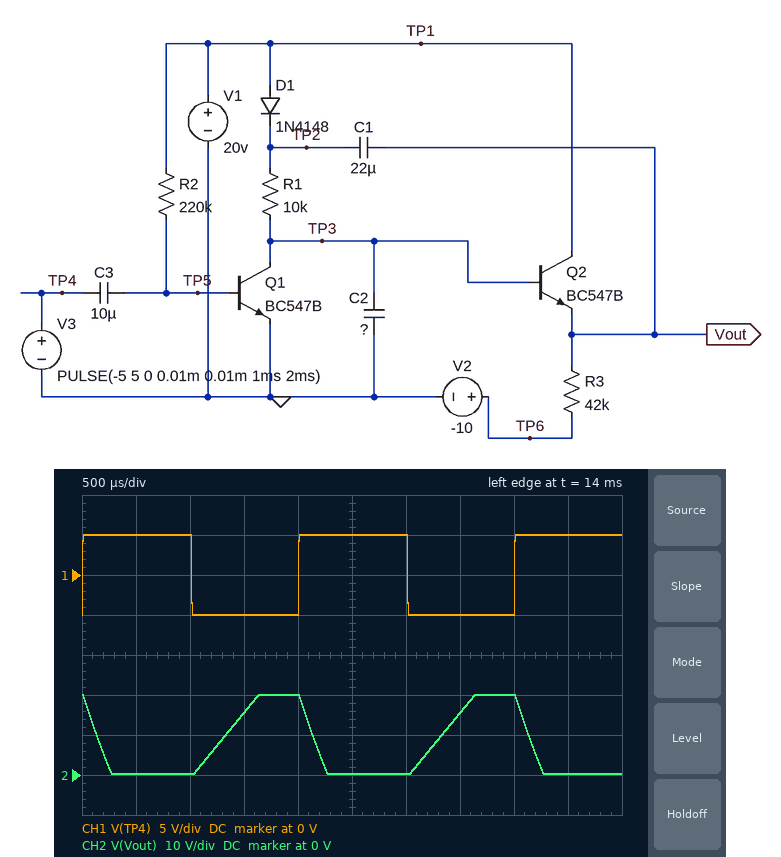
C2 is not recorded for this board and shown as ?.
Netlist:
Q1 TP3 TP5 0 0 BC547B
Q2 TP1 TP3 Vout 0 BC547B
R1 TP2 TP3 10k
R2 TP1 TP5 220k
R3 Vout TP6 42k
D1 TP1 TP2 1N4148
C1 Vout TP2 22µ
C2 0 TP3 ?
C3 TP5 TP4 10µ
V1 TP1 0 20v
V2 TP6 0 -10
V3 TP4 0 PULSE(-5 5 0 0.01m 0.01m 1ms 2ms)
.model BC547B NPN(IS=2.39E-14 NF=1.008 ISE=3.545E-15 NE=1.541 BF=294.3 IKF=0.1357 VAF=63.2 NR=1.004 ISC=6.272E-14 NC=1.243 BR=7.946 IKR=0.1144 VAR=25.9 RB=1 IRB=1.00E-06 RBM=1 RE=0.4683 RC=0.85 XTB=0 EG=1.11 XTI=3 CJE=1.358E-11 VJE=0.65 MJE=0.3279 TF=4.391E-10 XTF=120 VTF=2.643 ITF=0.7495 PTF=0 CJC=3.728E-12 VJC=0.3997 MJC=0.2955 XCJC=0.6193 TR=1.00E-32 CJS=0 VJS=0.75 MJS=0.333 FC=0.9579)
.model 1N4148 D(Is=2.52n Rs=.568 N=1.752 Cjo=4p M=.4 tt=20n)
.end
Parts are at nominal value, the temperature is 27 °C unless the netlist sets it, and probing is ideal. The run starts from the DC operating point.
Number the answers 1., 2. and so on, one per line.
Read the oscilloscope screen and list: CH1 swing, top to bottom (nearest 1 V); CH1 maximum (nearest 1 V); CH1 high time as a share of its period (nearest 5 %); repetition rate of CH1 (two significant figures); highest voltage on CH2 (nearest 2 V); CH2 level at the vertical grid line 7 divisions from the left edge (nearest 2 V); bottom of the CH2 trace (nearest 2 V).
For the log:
1. 10 V
2. 5 V
3. 50 %
4. 500 Hz
5. 20 V
6. 16 V
7. 0 V
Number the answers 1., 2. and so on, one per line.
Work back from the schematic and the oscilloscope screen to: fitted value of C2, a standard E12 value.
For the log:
1. 56 nF
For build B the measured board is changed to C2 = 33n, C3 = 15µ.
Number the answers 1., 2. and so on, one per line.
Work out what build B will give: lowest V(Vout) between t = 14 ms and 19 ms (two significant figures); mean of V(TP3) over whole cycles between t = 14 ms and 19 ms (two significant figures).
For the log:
1. 97 mV
2. 9.5 V
